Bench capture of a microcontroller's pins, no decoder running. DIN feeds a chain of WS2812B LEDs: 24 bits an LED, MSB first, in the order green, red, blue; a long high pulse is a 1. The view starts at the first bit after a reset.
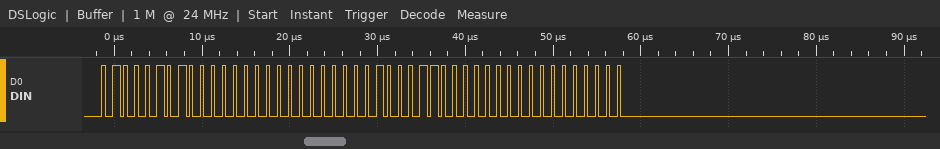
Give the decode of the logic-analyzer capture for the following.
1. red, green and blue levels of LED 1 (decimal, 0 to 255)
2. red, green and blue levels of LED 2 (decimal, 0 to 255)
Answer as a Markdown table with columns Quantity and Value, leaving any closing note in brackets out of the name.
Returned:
| Quantity | Value |
|---|---|
| red, green and blue levels of LED 1 | 0, 69, 0 |
| red, green and blue levels of LED 2 | 0, 70, 0 |
